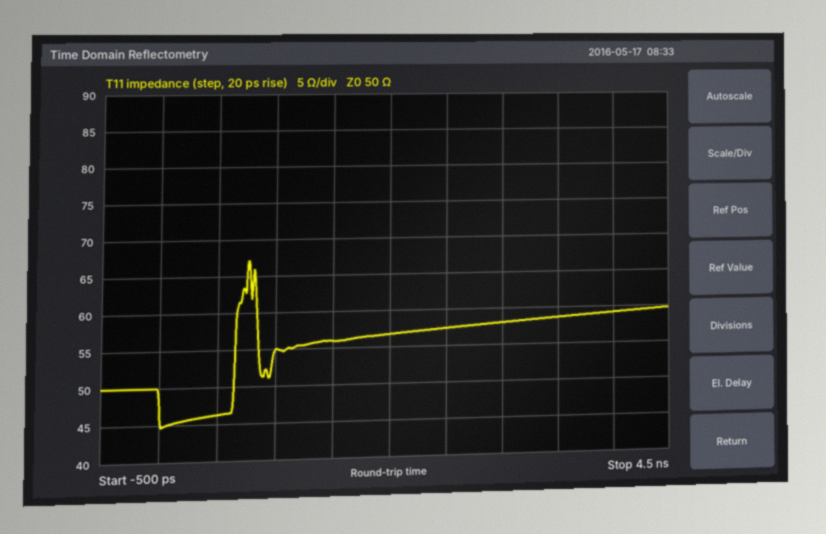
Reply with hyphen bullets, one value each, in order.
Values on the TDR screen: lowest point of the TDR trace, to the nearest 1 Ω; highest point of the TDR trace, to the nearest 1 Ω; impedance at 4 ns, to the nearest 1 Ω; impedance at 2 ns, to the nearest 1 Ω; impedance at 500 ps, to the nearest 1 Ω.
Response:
- 45 Ω
- 67 Ω
- 59 Ω
- 57 Ω
- 46 Ω
